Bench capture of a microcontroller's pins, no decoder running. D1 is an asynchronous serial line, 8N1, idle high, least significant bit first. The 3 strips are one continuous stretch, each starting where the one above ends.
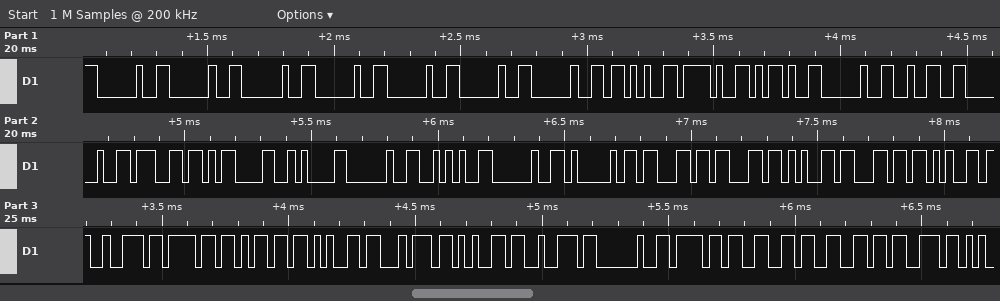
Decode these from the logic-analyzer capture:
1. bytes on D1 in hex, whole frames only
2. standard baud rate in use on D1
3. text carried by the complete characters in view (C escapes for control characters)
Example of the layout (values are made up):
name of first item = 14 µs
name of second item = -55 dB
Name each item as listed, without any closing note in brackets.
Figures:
bytes on D1 in hex, whole frames only = 20 20 20 20 20 20 20 2B 2F 2D 20 32 20 67 0D 0A 20 2A 20 41 63 63 65 6C 65 72 6F 6D 65 74 65 72 20 6F 66 66 73
standard baud rate in use on D1 = 38400 baud
text carried by the complete characters in view = "       +/- 2 g\r\n * Accelerometer offs"
